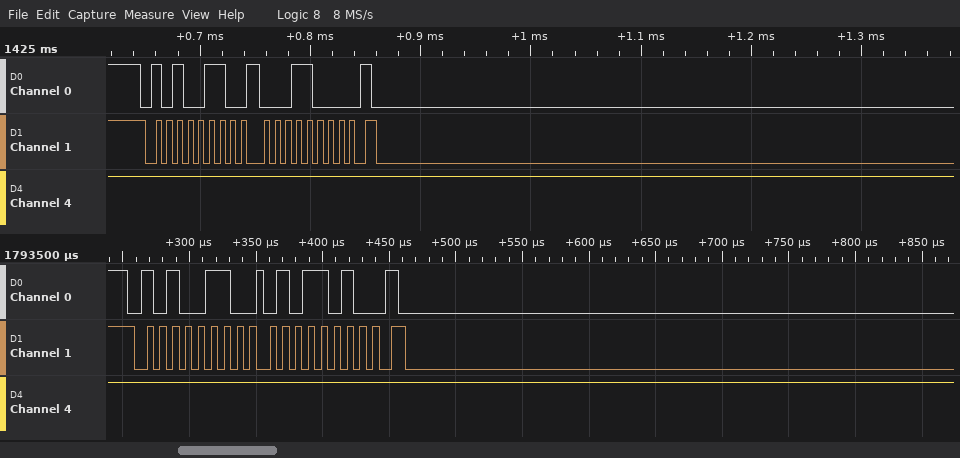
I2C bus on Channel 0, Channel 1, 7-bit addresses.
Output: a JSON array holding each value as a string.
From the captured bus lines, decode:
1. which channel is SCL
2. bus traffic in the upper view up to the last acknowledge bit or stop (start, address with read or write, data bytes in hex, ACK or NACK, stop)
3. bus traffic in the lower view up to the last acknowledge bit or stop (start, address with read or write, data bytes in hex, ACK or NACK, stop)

["Channel 1", "start, address 53 write ACK, 18 ACK", "start, address 53 write ACK, 5A ACK"]
